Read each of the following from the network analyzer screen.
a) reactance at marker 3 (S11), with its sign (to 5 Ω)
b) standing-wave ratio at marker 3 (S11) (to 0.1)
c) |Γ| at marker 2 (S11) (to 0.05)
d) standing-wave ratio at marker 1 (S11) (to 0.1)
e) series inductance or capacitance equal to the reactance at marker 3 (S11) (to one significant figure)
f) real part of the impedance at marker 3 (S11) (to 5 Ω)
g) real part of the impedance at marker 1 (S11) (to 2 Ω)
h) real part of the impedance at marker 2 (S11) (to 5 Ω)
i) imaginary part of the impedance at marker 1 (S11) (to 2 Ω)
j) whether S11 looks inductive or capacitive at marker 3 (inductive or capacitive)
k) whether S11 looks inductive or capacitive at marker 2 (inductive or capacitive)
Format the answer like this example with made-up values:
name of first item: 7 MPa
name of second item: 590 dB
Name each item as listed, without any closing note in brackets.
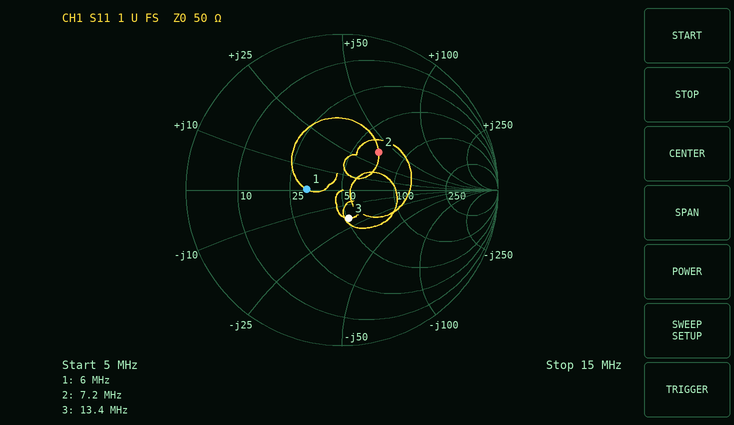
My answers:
reactance at marker 3 (S11), with its sign: -20 Ω
standing-wave ratio at marker 3 (S11): 1.5
|Γ| at marker 2 (S11): 0.35
standing-wave ratio at marker 1 (S11): 1.6
series inductance or capacitance equal to the reactance at marker 3 (S11): 600 pF
real part of the impedance at marker 3 (S11): 50 Ω
real part of the impedance at marker 1 (S11): 32 Ω
real part of the impedance at marker 2 (S11): 70 Ω
imaginary part of the impedance at marker 1 (S11): 0 Ω
whether S11 looks inductive or capacitive at marker 3: capacitive
whether S11 looks inductive or capacitive at marker 2: inductive
